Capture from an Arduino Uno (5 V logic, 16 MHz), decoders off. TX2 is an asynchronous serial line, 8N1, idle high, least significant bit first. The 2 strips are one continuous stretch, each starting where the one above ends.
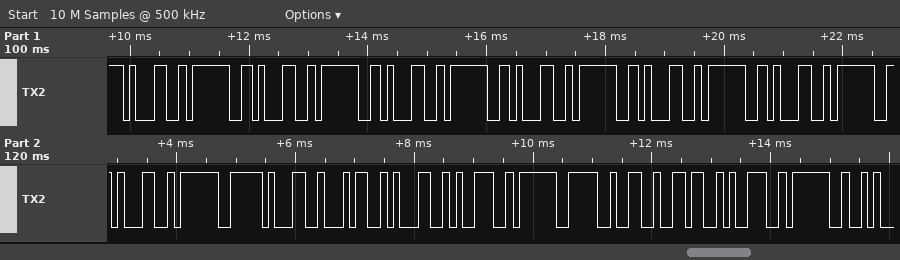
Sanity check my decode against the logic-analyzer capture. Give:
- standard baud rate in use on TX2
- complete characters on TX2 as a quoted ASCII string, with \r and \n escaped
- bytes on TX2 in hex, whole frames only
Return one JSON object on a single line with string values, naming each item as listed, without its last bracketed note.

{"standard baud rate in use on TX2": "9600 baud", "complete characters on TX2 as a quoted ASCII string, with \\r and \\n escaped": "\"1?1?1?1?1?1?1?1419?269?\"", "bytes on TX2 in hex, whole frames only": "31 3F 31 3F 31 3F 31 3F 31 3F 31 3F 31 3F 31 34 31 39 3F 32 36 39 3F"}
